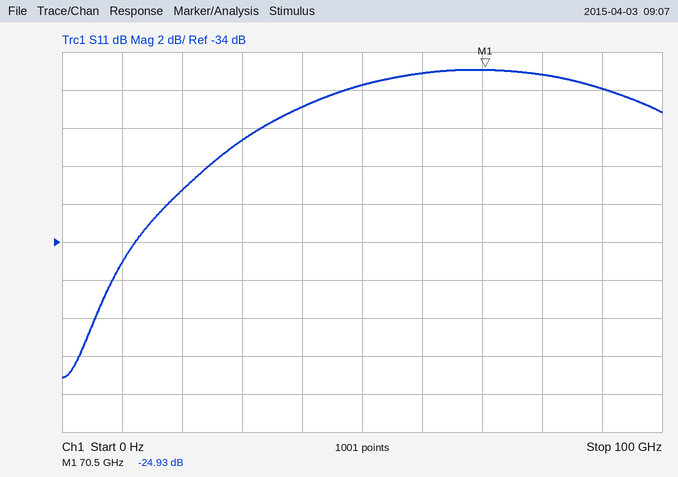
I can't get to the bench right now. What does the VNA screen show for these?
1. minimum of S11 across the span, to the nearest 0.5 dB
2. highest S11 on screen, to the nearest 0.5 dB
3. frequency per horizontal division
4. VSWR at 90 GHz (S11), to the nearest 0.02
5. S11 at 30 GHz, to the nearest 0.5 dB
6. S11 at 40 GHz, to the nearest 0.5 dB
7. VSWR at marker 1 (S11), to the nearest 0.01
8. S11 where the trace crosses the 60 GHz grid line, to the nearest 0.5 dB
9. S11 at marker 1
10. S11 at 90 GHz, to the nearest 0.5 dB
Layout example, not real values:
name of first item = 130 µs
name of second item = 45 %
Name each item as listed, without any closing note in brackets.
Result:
minimum of S11 across the span, to the nearest 0.5 dB = -41.0 dB
highest S11 on screen, to the nearest 0.5 dB = -25.0 dB
frequency per horizontal division = 10 GHz
VSWR at 90 GHz (S11), to the nearest 0.02 = 1.10
S11 at 30 GHz, to the nearest 0.5 dB = -28.5 dB
S11 at 40 GHz, to the nearest 0.5 dB = -27.0 dB
VSWR at marker 1 (S11), to the nearest 0.01 = 1.12
S11 where the trace crosses the 60 GHz grid line, to the nearest 0.5 dB = -25.0 dB
S11 at marker 1 = -24.93 dB
S11 at 90 GHz, to the nearest 0.5 dB = -26.0 dB
